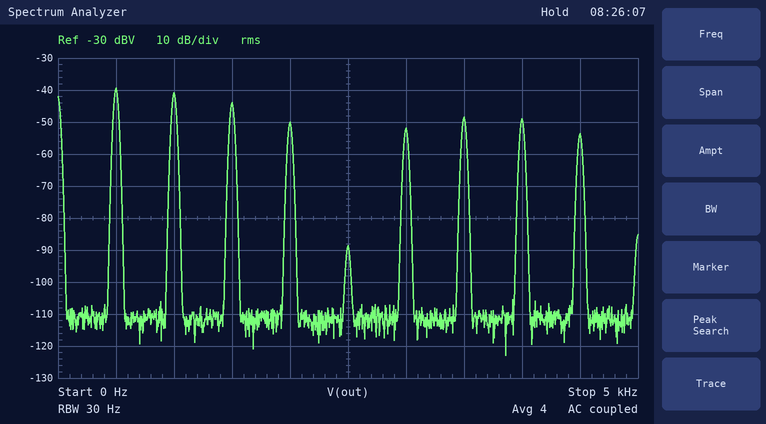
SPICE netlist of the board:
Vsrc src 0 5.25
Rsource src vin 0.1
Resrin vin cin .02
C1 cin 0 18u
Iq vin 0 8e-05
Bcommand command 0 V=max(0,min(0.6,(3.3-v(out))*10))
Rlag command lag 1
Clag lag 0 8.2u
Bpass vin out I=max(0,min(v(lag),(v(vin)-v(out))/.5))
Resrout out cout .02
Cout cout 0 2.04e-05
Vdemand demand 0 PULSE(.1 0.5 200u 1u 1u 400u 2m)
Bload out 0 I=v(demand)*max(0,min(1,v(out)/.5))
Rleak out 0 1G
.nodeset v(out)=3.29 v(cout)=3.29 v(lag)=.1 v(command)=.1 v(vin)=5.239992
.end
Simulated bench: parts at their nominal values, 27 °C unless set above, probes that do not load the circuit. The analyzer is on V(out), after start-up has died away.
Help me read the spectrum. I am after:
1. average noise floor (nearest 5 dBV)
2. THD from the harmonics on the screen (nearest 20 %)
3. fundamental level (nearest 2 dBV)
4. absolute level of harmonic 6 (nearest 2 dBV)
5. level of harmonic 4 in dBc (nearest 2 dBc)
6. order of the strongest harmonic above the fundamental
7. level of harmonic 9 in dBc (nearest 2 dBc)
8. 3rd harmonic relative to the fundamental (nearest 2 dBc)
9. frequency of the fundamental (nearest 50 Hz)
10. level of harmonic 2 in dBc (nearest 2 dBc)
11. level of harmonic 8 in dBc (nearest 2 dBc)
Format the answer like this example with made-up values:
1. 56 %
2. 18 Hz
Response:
1. -110 dBV
2. 120 %
3. -40 dBV
4. -52 dBV
5. -10 dBc
6. 2
7. -14 dBc
8. -4 dBc
9. 500 Hz
10. -2 dBc
11. -10 dBc
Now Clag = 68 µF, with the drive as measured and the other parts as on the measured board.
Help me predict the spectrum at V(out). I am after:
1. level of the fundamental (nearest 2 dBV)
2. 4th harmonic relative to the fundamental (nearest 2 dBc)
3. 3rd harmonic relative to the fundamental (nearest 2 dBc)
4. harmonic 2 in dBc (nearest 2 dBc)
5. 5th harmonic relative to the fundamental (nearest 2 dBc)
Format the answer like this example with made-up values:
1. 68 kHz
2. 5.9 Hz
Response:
1. -18 dBV
2. -4 dBc
3. 2 dBc
4. 4 dBc
5. -38 dBc
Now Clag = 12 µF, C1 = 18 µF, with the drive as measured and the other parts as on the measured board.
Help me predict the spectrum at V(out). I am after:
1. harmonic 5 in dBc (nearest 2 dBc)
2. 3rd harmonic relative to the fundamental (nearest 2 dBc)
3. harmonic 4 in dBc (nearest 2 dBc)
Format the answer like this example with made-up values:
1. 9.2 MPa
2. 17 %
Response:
1. -46 dBc
2. -2 dBc
3. -8 dBc
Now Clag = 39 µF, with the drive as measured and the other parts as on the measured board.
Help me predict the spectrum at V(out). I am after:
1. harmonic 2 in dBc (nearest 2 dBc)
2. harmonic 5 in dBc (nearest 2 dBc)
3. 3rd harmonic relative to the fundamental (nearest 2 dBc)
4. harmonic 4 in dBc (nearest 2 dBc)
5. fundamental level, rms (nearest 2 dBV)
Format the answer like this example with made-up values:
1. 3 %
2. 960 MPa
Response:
1. 4 dBc
2. -38 dBc
3. 4 dBc
4. -2 dBc
5. -26 dBV
